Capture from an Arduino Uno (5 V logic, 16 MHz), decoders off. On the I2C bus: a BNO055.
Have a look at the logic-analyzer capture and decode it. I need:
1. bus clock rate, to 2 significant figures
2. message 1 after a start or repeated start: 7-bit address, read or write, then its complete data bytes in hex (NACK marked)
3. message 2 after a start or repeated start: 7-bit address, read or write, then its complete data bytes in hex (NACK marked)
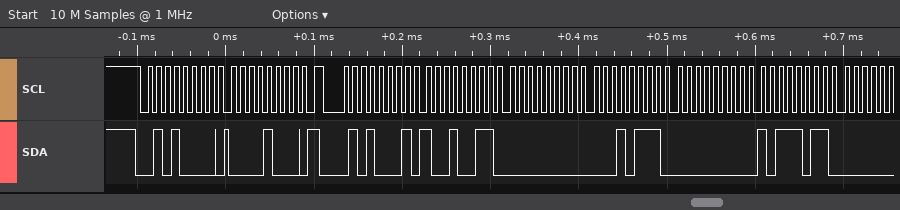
100 kHz
0x28 write: 08
0x28 read: 93 00 17 00 BB
